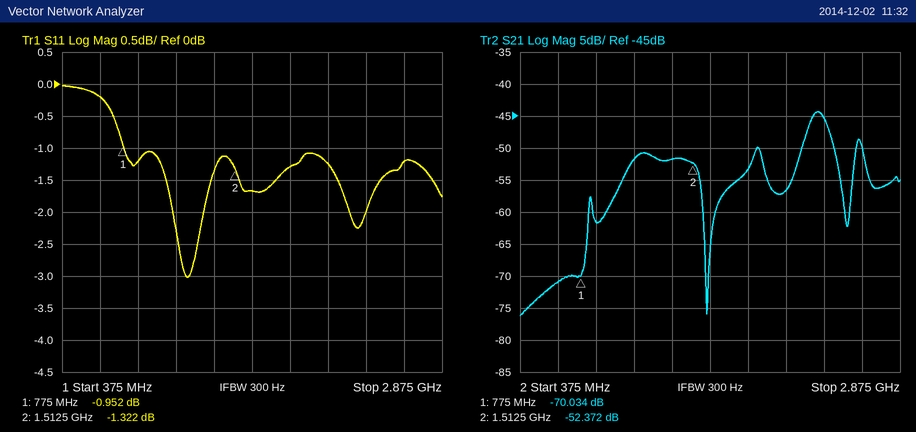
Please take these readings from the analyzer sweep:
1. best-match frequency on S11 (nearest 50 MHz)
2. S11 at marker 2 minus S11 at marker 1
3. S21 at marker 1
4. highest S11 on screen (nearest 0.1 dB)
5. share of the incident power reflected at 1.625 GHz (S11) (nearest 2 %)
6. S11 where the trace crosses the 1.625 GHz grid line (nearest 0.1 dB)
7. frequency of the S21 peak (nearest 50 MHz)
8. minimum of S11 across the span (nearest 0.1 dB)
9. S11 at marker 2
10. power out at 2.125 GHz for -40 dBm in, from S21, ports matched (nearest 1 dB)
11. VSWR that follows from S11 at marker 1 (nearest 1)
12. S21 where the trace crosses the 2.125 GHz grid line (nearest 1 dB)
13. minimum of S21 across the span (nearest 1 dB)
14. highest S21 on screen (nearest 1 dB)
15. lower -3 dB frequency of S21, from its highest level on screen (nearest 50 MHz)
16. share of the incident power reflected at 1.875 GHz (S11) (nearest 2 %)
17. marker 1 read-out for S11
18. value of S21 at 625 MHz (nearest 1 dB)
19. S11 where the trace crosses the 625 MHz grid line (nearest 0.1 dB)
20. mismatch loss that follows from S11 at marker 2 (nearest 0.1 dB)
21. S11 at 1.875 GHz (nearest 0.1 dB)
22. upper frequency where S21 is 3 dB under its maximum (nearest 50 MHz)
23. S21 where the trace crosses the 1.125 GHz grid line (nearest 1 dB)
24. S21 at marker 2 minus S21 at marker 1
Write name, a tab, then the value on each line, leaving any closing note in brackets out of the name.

best-match frequency on S11	1.20 GHz
S11 at marker 2 minus S11 at marker 1	-0.370 dB
S21 at marker 1	-70.034 dB
highest S11 on screen	0.0 dB
share of the incident power reflected at 1.625 GHz (S11)	68 %
S11 where the trace crosses the 1.625 GHz grid line	-1.7 dB
frequency of the S21 peak	2.35 GHz
minimum of S11 across the span	-3.0 dB
S11 at marker 2	-1.322 dB
power out at 2.125 GHz for -40 dBm in, from S21, ports matched	-97 dBm
VSWR that follows from S11 at marker 1	18
S21 where the trace crosses the 2.125 GHz grid line	-57 dB
minimum of S21 across the span	-76 dB
highest S21 on screen	-44 dB
lower -3 dB frequency of S21, from its highest level on screen	2.25 GHz
share of the incident power reflected at 1.875 GHz (S11)	74 %
marker 1 read-out for S11	-0.952 dB
value of S21 at 625 MHz	-71 dB
S11 where the trace crosses the 625 MHz grid line	-0.2 dB
mismatch loss that follows from S11 at marker 2	5.8 dB
S11 at 1.875 GHz	-1.3 dB
upper frequency where S21 is 3 dB under its maximum	2.40 GHz
S21 where the trace crosses the 1.125 GHz grid line	-52 dB
S21 at marker 2 minus S21 at marker 1	17.662 dB
